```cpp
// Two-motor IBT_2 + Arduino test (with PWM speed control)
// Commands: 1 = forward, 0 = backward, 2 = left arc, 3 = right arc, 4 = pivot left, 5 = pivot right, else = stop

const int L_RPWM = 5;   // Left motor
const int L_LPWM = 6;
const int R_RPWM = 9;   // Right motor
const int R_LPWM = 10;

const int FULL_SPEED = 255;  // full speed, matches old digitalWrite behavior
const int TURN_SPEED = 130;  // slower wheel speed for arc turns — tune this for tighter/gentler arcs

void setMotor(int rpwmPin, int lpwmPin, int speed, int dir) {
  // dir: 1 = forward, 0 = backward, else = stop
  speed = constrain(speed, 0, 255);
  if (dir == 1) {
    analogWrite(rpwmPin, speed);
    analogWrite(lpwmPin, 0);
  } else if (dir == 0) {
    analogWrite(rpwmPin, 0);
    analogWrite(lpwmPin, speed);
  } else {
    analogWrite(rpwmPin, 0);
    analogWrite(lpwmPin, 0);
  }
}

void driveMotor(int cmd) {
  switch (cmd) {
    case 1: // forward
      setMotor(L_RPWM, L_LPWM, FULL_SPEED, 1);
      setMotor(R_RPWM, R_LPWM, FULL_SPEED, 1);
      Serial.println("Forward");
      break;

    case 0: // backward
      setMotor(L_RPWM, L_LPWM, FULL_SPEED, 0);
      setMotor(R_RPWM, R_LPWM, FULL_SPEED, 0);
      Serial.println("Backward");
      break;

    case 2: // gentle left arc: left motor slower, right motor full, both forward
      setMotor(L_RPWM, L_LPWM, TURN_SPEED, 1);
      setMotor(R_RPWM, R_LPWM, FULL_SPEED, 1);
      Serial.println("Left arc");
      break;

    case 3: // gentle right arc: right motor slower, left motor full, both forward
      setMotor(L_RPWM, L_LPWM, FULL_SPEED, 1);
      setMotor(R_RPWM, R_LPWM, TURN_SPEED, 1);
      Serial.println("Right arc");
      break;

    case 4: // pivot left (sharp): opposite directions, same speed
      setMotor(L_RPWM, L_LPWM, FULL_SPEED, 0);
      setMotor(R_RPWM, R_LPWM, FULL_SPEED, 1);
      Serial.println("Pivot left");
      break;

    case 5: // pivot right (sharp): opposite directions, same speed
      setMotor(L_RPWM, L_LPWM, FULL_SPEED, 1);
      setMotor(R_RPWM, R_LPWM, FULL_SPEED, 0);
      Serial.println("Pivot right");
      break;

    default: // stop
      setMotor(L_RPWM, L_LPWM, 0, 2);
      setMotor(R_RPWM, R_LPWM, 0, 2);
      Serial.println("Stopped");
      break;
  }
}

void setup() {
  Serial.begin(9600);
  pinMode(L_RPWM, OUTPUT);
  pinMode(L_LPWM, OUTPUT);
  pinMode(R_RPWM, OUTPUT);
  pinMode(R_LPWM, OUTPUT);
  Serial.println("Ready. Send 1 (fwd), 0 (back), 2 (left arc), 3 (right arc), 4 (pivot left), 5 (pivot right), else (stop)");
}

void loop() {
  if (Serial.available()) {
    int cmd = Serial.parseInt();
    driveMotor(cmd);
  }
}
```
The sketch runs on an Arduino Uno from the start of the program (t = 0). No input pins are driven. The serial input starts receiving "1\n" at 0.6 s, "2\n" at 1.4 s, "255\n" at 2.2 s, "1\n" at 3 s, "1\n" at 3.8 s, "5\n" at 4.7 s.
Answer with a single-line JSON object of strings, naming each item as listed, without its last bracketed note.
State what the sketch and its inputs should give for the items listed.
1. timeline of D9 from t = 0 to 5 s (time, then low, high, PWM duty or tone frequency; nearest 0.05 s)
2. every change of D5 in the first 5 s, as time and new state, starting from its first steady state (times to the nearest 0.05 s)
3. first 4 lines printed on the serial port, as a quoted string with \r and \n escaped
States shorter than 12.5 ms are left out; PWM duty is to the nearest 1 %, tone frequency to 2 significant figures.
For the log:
{"timeline of D9 from t = 0 to 5 s": "0 s low; 0.6 s high; 2.2 s low; 3 s high; 4.7 s low", "every change of D5 in the first 5 s, as time and new state, starting from its first steady state": "0 s low; 0.6 s high; 1.4 s PWM 51 %; 2.2 s low; 3 s high", "first 4 lines printed on the serial port, as a quoted string with \\r and \\n escaped": "\"Ready. Send 1 (fwd), 0 (back), 2 (left arc), 3 (right arc), 4 (pivot left), 5 (pivot right), else (stop)\\r\\nForward\\r\\nLeft arc\\r\\nStopped\\r\\n\""}
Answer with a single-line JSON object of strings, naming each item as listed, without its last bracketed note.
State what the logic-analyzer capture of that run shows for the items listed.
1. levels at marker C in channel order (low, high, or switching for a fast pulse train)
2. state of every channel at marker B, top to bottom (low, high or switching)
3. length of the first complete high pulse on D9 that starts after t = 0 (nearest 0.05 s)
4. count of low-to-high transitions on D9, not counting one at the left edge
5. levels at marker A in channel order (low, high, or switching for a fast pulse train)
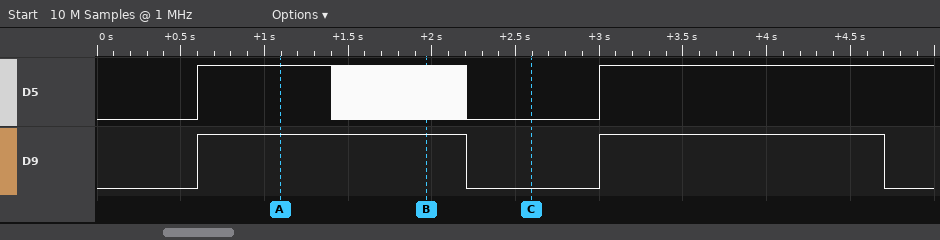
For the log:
{"levels at marker C in channel order": "D5 low, D9 low", "state of every channel at marker B, top to bottom": "D5 switching, D9 high", "length of the first complete high pulse on D9 that starts after t = 0": "1.60 s", "count of low-to-high transitions on D9, not counting one at the left edge": "2", "levels at marker A in channel order": "D5 high, D9 high"}
